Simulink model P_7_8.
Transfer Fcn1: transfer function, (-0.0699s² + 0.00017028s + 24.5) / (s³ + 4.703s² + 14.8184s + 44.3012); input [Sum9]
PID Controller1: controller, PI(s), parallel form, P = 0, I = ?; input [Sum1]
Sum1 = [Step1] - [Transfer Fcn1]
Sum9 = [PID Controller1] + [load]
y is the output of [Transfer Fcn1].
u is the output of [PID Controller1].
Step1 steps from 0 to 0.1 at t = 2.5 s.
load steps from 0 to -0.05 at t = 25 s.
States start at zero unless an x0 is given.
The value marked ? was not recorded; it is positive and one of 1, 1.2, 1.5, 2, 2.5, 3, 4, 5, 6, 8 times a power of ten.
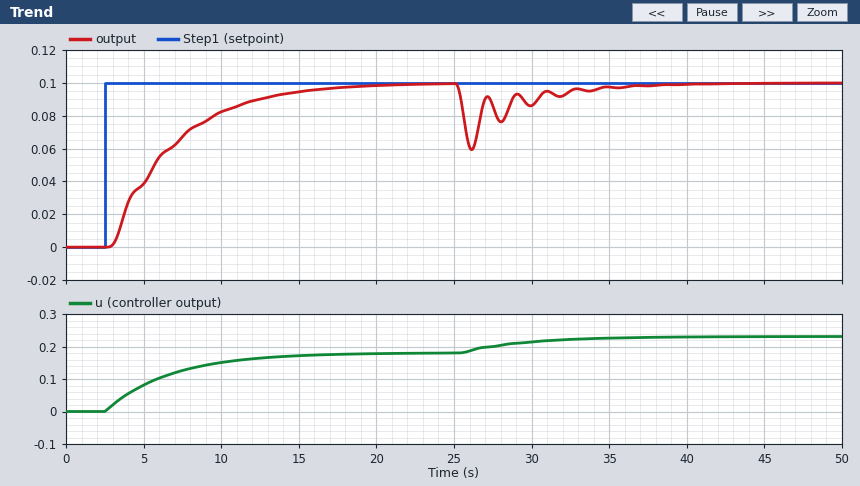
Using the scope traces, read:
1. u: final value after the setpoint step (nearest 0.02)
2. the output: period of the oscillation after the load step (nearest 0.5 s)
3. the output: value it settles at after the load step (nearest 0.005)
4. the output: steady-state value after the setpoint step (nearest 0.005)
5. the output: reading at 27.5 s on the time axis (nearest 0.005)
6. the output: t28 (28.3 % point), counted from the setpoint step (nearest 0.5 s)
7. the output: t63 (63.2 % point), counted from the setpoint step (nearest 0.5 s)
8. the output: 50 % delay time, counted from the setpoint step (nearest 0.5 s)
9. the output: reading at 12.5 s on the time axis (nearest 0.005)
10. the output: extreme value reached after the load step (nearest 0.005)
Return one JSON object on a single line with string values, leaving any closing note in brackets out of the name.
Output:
{"u: final value after the setpoint step": "0.18", "the output: period of the oscillation after the load step": "2.0 s", "the output: value it settles at after the load step": "0.100", "the output: steady-state value after the setpoint step": "0.100", "the output: reading at 27.5 s on the time axis": "0.085", "the output: t28 (28.3 % point), counted from the setpoint step": "1.5 s", "the output: t63 (63.2 % point), counted from the setpoint step": "4.5 s", "the output: 50 % delay time, counted from the setpoint step": "3.0 s", "the output: reading at 12.5 s on the time axis": "0.090", "the output: extreme value reached after the load step": "0.060"}
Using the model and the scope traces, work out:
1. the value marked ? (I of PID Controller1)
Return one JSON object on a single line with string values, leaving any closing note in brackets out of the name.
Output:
{"the value marked ?": "0.4"}
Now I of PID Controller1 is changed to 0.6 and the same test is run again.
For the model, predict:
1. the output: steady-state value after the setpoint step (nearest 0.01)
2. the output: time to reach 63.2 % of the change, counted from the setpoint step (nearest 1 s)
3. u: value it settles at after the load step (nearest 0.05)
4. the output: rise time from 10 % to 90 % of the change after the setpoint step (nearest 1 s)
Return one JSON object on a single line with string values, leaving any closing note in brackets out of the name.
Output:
{"the output: steady-state value after the setpoint step": "0.10", "the output: time to reach 63.2 % of the change, counted from the setpoint step": "3 s", "u: value it settles at after the load step": "0.25", "the output: rise time from 10 % to 90 % of the change after the setpoint step": "6 s"}
